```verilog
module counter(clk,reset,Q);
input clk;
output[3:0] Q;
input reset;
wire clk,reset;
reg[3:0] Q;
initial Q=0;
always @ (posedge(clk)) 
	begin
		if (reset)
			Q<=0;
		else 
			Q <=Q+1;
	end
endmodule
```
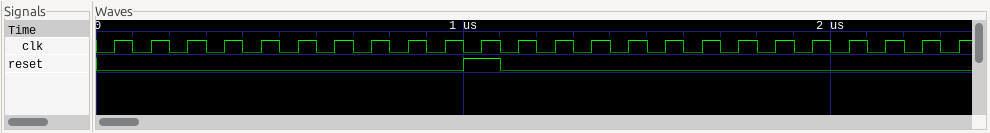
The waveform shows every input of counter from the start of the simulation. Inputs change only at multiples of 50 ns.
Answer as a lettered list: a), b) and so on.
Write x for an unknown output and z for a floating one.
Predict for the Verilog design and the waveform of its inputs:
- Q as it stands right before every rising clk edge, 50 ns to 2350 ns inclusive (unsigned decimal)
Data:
a) 0, 1, 2, 3, 4, 5, 6, 7, 8, 9, 10, 0, 1, 2, 3, 4, 5, 6, 7, 8, 9, 10, 11, 12
